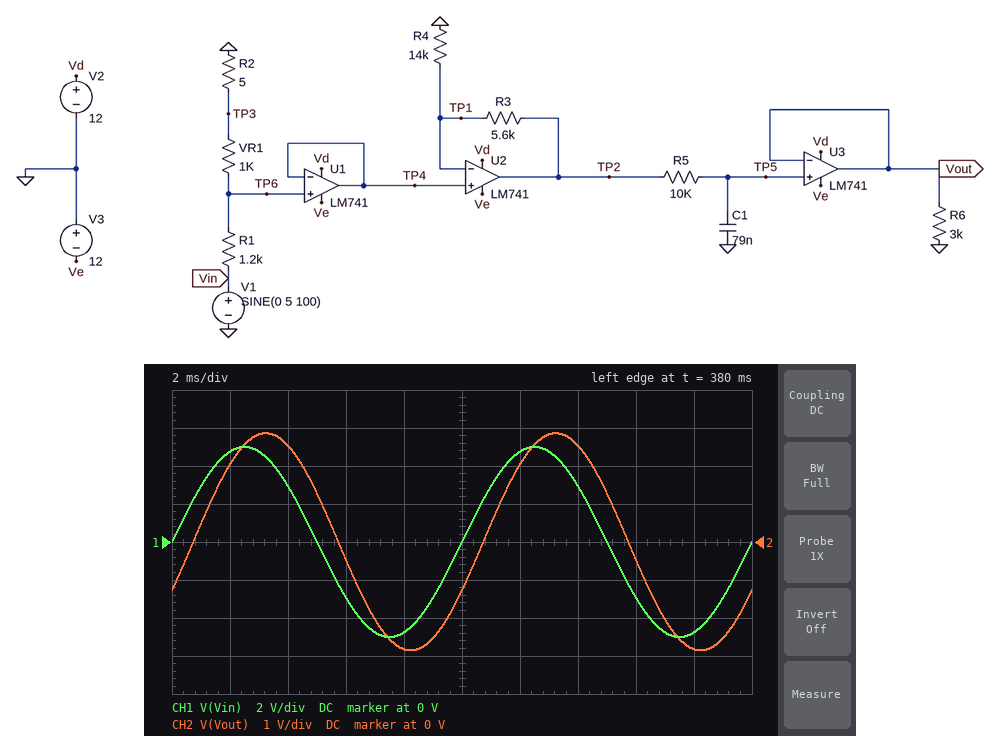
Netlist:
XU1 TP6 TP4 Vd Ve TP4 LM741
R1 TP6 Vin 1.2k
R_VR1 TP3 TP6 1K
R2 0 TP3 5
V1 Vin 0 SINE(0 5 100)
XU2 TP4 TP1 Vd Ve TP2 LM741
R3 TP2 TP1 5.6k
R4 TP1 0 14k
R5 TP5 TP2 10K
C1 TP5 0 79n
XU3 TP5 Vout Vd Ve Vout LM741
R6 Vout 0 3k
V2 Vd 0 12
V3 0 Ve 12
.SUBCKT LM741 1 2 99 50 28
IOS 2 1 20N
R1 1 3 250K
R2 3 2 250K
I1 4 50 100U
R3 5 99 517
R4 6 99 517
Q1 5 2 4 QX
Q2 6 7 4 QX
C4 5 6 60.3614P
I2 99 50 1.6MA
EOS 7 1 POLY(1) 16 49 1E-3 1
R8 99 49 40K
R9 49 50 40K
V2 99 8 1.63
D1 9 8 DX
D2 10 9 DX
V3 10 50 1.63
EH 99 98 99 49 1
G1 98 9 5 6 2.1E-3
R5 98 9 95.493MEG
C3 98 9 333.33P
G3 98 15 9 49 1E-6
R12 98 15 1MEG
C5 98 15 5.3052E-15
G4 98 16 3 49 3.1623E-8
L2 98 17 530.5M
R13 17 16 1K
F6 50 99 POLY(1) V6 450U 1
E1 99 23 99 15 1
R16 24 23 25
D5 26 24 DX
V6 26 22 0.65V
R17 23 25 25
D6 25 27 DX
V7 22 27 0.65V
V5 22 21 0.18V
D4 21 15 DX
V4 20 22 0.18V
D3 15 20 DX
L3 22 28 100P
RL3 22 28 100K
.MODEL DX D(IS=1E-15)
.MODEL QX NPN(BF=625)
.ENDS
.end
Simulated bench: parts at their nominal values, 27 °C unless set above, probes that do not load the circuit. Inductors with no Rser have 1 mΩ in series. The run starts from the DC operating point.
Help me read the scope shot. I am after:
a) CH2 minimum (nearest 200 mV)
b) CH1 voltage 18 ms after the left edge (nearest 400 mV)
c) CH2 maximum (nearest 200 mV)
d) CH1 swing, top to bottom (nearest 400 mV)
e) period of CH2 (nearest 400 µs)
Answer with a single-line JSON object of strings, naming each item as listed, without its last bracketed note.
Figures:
{"CH2 minimum": "-2.8 V", "CH1 voltage 18 ms after the left edge": "-4.8 V", "CH2 maximum": "2.8 V", "CH1 swing, top to bottom": "10.0 V", "period of CH2": "10.0 ms"}
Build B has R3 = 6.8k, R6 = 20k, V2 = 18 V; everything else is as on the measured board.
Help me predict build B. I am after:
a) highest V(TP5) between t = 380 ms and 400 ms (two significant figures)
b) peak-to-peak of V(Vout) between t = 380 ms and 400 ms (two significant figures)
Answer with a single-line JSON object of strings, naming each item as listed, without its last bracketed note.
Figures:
{"highest V(TP5) between t = 380 ms and 400 ms": "3.0 V", "peak-to-peak of V(Vout) between t = 380 ms and 400 ms": "6.1 V"}
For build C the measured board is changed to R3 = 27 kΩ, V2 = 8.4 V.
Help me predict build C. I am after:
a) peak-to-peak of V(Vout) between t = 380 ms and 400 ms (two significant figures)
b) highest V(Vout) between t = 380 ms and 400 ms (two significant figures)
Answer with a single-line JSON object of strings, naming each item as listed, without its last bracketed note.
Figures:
{"peak-to-peak of V(Vout) between t = 380 ms and 400 ms": "12 V", "highest V(Vout) between t = 380 ms and 400 ms": "6.0 V"}
